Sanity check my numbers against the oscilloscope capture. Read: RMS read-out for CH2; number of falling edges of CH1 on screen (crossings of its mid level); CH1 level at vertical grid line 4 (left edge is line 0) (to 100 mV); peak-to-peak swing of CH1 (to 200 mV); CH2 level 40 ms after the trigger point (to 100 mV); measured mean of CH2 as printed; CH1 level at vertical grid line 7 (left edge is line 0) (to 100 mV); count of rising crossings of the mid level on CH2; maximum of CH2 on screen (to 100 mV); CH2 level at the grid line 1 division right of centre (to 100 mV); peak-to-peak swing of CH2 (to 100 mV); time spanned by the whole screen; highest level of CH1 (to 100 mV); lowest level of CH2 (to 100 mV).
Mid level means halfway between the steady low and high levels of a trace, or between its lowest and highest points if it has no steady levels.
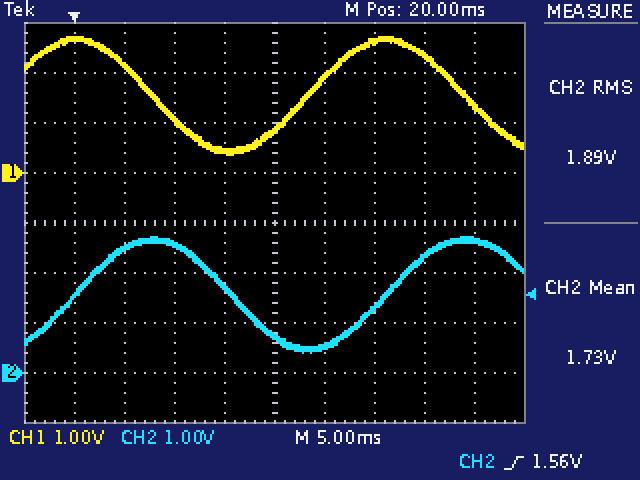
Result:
1.89 V
2
400 mV
2.4 V
2.7 V
1.73 V
2.6 V
2
2.7 V
500 mV
2.3 V
50 ms
2.7 V
400 mV
